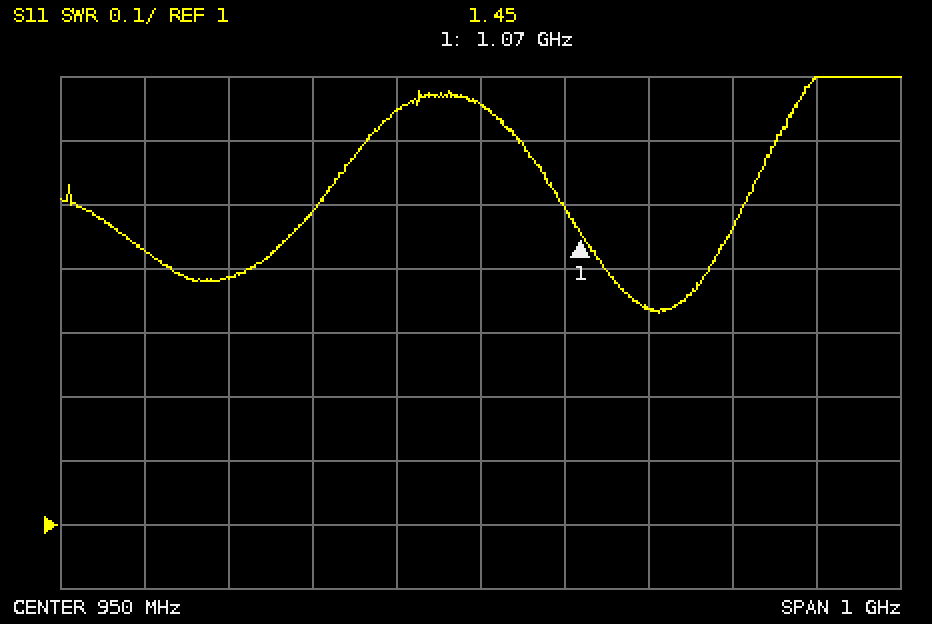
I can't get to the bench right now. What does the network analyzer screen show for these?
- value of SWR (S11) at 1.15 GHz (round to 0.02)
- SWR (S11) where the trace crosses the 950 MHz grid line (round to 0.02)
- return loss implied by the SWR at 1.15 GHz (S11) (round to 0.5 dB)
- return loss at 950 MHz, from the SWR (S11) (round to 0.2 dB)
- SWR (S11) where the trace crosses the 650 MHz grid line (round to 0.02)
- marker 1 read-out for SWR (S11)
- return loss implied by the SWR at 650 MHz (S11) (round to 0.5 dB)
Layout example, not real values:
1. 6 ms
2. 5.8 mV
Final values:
1. 1.34
2. 1.66
3. 17.0 dB
4. 12.2 dB
5. 1.38
6. 1.45
7. 16.0 dB
